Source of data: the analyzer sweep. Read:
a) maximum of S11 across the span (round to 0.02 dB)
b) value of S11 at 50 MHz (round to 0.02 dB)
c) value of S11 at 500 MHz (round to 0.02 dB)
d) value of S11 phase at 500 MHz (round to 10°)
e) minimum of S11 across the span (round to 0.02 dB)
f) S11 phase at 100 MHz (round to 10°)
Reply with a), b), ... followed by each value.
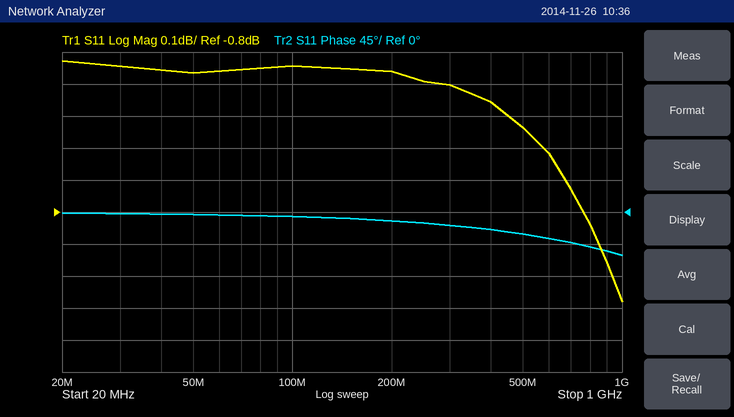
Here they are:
a) -0.32 dB
b) -0.36 dB
c) -0.54 dB
d) -30°
e) -1.08 dB
f) -10°
